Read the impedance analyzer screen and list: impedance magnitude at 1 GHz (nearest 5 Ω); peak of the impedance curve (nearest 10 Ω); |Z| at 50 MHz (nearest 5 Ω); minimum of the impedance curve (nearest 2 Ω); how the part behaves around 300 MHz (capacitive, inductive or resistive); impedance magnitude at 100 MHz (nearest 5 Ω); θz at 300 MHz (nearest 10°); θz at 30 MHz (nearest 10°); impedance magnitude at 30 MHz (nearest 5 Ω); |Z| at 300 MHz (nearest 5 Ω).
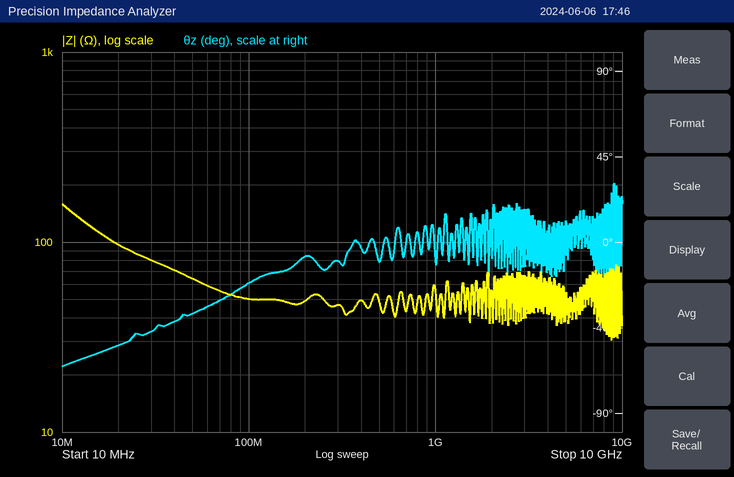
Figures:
55 Ω
160 Ω
65 Ω
30 Ω
resistive
50 Ω
-10°
-50°
80 Ω
45 Ω
